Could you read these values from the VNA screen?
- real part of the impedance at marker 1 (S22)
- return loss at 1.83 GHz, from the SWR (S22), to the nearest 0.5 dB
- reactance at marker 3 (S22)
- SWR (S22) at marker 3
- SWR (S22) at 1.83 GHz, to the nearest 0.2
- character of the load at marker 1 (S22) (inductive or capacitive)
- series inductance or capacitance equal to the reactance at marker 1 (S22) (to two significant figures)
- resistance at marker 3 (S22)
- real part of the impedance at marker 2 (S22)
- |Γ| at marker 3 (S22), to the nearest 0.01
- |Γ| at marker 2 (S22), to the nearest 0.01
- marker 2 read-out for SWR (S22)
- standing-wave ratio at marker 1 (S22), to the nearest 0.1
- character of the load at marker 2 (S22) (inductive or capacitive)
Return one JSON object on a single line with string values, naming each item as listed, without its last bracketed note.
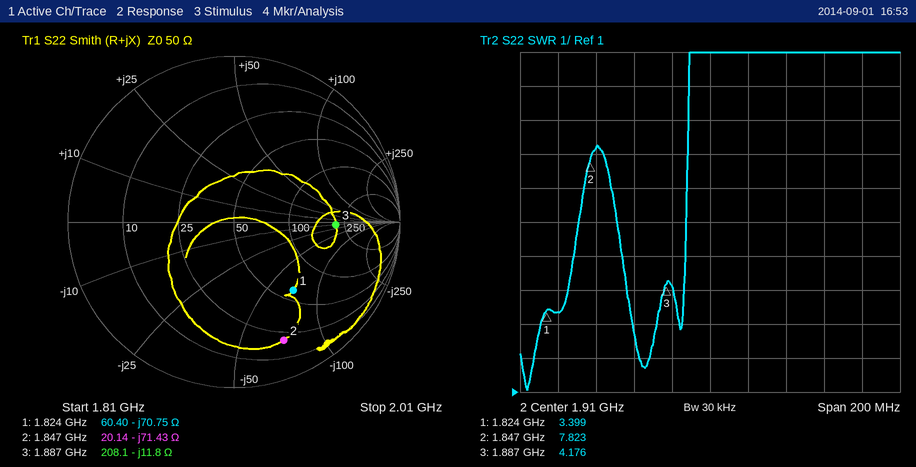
{"real part of the impedance at marker 1": "60.40 Ω", "return loss at 1.83 GHz, from the SWR (S22), to the nearest 0.5 dB": "5.5 dB", "reactance at marker 3": "-11.8 Ω", "SWR (S22) at marker 3": "4.176", "SWR (S22) at 1.83 GHz, to the nearest 0.2": "3.4", "character of the load at marker 1 (S22)": "capacitive", "series inductance or capacitance equal to the reactance at marker 1 (S22)": "1.2 pF", "resistance at marker 3": "208.1 Ω", "real part of the impedance at marker 2": "20.14 Ω", "|Γ| at marker 3 (S22), to the nearest 0.01": "0.61", "|Γ| at marker 2 (S22), to the nearest 0.01": "0.77", "marker 2 read-out for SWR": "7.823", "standing-wave ratio at marker 1 (S22), to the nearest 0.1": "3.4", "character of the load at marker 2 (S22)": "capacitive"}
